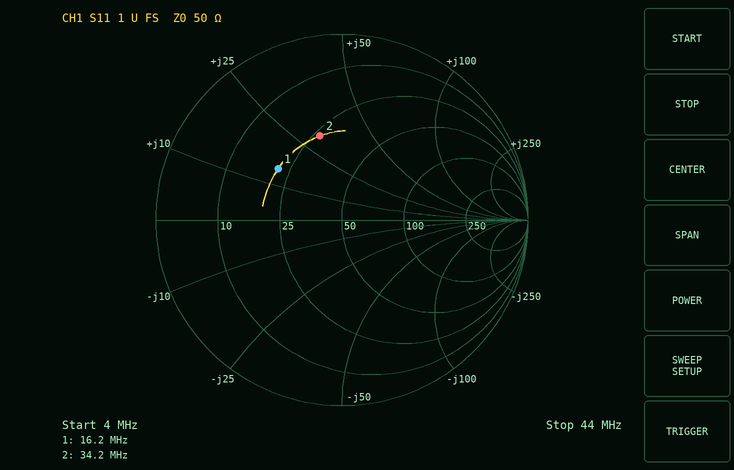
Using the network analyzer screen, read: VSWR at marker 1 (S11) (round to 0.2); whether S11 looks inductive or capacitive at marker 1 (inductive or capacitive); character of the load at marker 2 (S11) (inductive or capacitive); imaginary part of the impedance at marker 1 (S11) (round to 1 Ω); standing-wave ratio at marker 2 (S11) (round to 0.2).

2.6
inductive
inductive
+15 Ω
2.8
